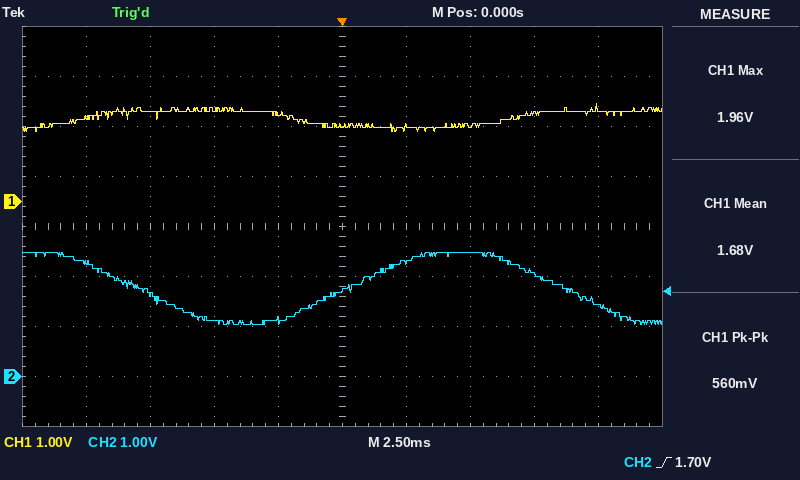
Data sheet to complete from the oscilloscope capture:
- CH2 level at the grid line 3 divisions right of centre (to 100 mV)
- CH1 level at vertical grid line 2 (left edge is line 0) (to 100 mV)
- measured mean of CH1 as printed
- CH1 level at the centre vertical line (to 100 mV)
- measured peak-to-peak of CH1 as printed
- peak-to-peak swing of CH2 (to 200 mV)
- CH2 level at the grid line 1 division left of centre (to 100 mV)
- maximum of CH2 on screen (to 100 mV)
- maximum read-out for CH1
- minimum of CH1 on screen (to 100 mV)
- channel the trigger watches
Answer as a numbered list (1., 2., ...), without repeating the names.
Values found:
1. 2.0 V
2. 1.8 V
3. 1.68 V
4. 1.5 V
5. 560 mV
6. 1.4 V
7. 1.1 V
8. 2.5 V
9. 1.96 V
10. 1.4 V
11. CH2
